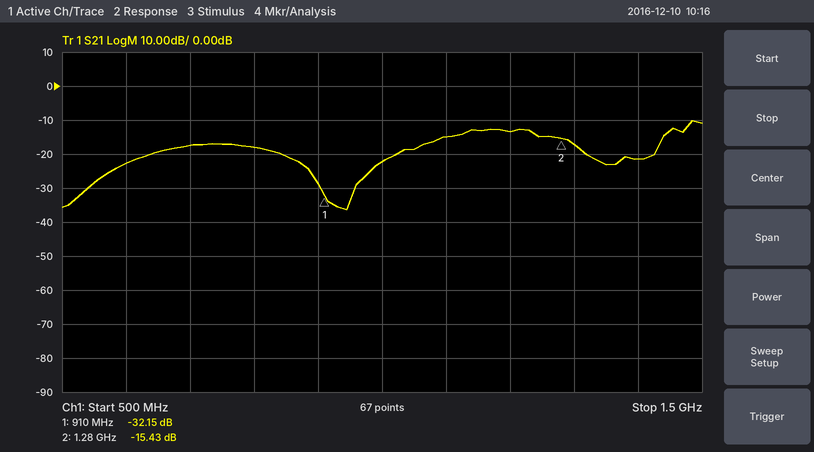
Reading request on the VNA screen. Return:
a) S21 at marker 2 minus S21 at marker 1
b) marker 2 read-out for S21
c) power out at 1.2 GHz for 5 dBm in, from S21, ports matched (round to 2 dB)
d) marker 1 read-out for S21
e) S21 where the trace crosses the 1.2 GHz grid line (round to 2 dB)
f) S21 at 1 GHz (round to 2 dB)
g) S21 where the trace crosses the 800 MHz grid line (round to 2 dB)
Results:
16.72 dB
-15.43 dB
-8 dBm
-32.15 dB
-14 dB
-22 dB
-18 dB
